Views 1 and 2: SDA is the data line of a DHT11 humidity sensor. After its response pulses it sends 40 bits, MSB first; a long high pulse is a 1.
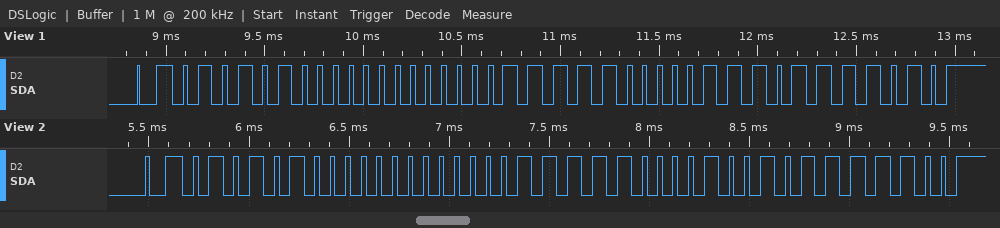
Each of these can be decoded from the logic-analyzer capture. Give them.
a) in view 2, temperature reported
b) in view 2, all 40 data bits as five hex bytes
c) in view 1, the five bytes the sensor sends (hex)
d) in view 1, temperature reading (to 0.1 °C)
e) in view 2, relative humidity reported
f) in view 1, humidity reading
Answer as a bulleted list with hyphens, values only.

- 31.9 °C
- 54 00 1F 09 7C
- 54 00 1F 07 7A
- 31.7 °C
- 84 %
- 84 %
